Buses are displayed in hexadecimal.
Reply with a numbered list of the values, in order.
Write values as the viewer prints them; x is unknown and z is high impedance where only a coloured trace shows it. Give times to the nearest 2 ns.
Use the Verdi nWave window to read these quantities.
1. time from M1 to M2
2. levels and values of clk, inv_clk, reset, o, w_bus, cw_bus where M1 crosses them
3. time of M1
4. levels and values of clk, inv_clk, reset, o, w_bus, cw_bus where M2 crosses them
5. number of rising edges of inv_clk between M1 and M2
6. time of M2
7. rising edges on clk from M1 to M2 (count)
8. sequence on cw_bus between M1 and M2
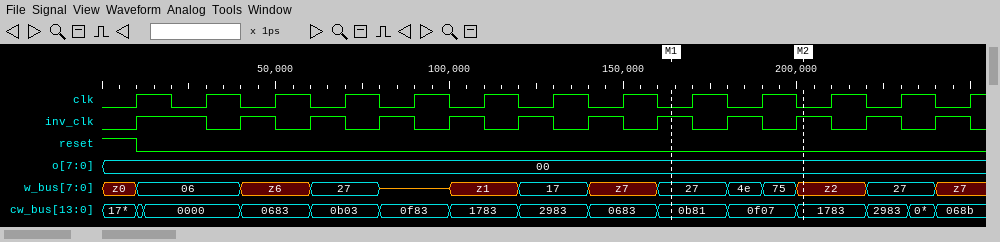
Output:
1. 38 ns
2. clk=0, inv_clk=1, reset=0, o=00, w_bus=27, cw_bus=0b81
3. 164 ns
4. clk=0, inv_clk=1, reset=0, o=00, w_bus=z2, cw_bus=1783
5. 2
6. 202 ns
7. 2
8. 0b81, 0f07, 1783
